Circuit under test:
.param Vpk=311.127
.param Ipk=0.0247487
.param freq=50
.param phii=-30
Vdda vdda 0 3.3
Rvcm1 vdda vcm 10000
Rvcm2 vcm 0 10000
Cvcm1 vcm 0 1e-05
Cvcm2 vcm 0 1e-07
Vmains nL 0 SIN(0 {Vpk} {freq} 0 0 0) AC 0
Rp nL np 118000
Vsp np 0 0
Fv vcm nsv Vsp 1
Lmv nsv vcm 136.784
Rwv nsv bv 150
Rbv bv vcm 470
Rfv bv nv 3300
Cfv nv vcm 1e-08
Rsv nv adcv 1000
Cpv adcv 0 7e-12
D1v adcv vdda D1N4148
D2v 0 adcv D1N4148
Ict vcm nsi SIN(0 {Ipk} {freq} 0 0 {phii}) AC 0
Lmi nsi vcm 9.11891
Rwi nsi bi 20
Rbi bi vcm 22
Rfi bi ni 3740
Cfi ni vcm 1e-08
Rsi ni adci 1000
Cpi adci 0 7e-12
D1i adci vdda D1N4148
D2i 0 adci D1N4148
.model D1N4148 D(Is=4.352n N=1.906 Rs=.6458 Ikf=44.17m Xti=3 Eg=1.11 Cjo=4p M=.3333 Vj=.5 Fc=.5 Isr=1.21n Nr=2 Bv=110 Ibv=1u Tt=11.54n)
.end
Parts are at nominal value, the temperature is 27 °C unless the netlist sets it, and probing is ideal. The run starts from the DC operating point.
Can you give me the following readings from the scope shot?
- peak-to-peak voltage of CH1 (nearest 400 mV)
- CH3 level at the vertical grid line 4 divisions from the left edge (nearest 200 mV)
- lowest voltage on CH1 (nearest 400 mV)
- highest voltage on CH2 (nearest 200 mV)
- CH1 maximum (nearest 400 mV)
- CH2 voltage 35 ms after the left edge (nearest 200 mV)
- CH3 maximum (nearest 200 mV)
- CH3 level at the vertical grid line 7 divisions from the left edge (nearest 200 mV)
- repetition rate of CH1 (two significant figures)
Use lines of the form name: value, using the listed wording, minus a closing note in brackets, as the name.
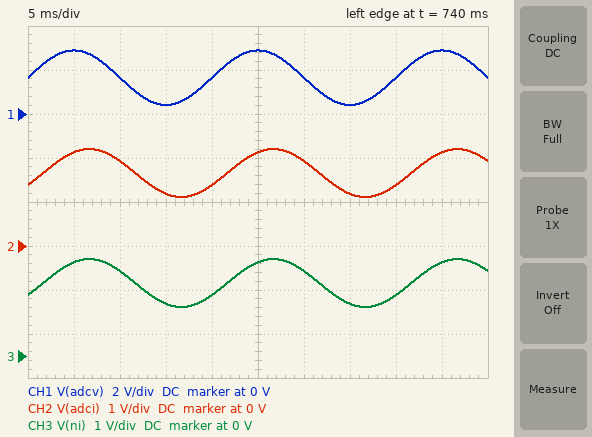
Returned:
peak-to-peak voltage of CH1: 2.4 V
CH3 level at the vertical grid line 4 divisions from the left edge: 1.4 V
lowest voltage on CH1: 400 mV
highest voltage on CH2: 2.2 V
CH1 maximum: 2.8 V
CH2 voltage 35 ms after the left edge: 1.2 V
CH3 maximum: 2.2 V
CH3 level at the vertical grid line 7 divisions from the left edge: 1.2 V
repetition rate of CH1: 50 Hz
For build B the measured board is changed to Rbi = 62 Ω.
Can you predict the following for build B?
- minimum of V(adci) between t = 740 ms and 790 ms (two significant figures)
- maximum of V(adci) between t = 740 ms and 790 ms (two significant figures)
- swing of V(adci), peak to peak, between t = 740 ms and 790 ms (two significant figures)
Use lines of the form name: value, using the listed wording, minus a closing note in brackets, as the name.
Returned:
minimum of V(adci) between t = 740 ms and 790 ms: 120 mV
maximum of V(adci) between t = 740 ms and 790 ms: 3.2 V
swing of V(adci), peak to peak, between t = 740 ms and 790 ms: 3.1 V
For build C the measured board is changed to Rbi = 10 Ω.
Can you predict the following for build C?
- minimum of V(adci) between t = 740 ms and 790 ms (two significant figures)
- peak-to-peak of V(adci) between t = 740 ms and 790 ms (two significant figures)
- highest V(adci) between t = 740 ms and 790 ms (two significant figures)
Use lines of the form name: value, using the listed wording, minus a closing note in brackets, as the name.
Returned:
minimum of V(adci) between t = 740 ms and 790 ms: 1.4 V
peak-to-peak of V(adci) between t = 740 ms and 790 ms: 500 mV
highest V(adci) between t = 740 ms and 790 ms: 1.9 V
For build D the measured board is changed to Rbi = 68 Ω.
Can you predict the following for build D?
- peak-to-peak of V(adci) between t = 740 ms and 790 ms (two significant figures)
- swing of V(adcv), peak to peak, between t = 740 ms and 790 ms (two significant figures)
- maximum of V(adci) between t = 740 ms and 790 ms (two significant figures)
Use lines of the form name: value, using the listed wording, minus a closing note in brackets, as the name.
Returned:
peak-to-peak of V(adci) between t = 740 ms and 790 ms: 3.4 V
swing of V(adcv), peak to peak, between t = 740 ms and 790 ms: 2.5 V
maximum of V(adci) between t = 740 ms and 790 ms: 3.3 V
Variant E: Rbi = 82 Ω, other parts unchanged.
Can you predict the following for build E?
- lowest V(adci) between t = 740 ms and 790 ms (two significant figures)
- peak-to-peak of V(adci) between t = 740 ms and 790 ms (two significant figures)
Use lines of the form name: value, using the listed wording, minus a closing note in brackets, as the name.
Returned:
lowest V(adci) between t = 740 ms and 790 ms: -350 mV
peak-to-peak of V(adci) between t = 740 ms and 790 ms: 4.0 V
